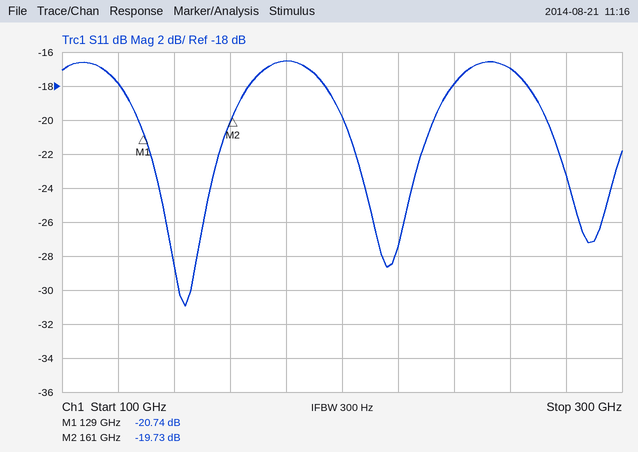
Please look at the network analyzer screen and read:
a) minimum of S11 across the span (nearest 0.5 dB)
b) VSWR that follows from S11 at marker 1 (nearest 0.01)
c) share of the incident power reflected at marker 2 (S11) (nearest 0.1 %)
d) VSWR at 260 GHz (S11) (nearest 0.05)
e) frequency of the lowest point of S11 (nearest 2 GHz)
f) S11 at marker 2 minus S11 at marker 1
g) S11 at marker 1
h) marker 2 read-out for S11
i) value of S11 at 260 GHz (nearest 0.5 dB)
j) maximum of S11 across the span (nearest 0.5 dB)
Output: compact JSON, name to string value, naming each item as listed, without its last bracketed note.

{"minimum of S11 across the span": "-31.0 dB", "VSWR that follows from S11 at marker 1": "1.20", "share of the incident power reflected at marker 2 (S11)": "1.1 %", "VSWR at 260 GHz (S11)": "1.35", "frequency of the lowest point of S11": "144 GHz", "S11 at marker 2 minus S11 at marker 1": "1.01 dB", "S11 at marker 1": "-20.74 dB", "marker 2 read-out for S11": "-19.73 dB", "value of S11 at 260 GHz": "-17.0 dB", "maximum of S11 across the span": "-16.5 dB"}
